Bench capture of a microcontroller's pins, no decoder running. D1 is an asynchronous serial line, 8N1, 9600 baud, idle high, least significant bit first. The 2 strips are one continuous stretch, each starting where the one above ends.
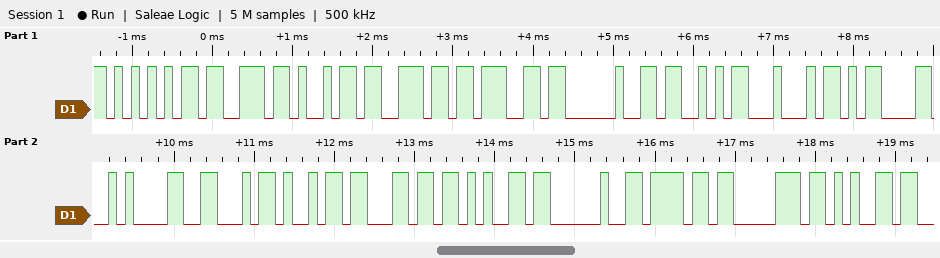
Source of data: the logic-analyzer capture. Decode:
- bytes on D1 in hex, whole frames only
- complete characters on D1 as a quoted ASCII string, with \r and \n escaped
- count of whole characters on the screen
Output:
0x55 0x73 0x69 0x6E 0x67 0x20 0x53 0x44 0x0D 0x0A 0x46 0x69 0x6C 0x65 0x20 0x6F 0x70 0x65
"Using SD\r\nFile ope"
18
